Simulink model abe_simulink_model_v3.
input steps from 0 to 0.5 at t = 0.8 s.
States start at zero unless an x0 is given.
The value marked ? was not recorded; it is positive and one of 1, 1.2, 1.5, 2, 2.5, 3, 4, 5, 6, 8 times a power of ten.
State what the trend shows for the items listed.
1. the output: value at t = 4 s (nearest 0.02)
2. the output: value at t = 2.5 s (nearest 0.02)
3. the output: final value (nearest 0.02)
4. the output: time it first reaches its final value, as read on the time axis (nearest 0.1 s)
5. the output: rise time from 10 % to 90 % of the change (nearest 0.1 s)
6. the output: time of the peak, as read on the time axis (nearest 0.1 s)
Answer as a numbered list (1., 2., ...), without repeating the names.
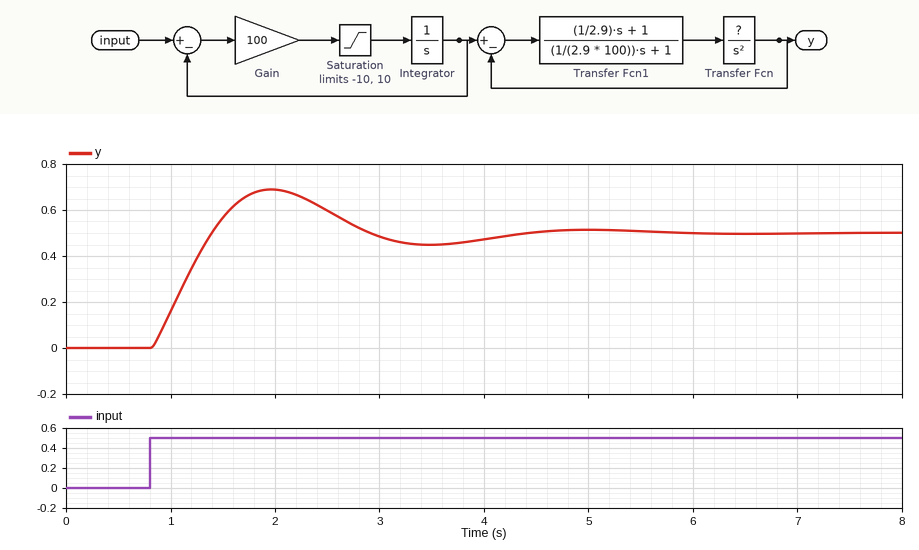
1. 0.48
2. 0.60
3. 0.50
4. 1.4 s
5. 0.4 s
6. 2.0 s
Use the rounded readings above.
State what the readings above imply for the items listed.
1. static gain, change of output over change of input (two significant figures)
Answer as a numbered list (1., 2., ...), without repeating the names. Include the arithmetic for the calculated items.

1. (0.5 - 0) / (0.5 - 0) = 1.0
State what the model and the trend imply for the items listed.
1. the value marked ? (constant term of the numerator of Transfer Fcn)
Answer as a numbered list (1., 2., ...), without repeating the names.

1. 5
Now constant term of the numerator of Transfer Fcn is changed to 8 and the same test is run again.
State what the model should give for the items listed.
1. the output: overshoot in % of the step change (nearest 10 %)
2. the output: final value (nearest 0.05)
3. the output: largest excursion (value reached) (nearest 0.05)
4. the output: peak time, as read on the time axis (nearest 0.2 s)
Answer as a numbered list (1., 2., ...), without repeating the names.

1. 30 %
2. 0.50
3. 0.65
4. 1.6 s
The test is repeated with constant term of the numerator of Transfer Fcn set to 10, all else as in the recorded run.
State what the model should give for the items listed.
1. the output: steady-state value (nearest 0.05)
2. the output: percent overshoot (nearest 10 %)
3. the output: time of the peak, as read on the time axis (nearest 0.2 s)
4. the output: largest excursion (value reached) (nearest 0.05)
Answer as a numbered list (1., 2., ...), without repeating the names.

1. 0.50
2. 30 %
3. 1.6 s
4. 0.65
